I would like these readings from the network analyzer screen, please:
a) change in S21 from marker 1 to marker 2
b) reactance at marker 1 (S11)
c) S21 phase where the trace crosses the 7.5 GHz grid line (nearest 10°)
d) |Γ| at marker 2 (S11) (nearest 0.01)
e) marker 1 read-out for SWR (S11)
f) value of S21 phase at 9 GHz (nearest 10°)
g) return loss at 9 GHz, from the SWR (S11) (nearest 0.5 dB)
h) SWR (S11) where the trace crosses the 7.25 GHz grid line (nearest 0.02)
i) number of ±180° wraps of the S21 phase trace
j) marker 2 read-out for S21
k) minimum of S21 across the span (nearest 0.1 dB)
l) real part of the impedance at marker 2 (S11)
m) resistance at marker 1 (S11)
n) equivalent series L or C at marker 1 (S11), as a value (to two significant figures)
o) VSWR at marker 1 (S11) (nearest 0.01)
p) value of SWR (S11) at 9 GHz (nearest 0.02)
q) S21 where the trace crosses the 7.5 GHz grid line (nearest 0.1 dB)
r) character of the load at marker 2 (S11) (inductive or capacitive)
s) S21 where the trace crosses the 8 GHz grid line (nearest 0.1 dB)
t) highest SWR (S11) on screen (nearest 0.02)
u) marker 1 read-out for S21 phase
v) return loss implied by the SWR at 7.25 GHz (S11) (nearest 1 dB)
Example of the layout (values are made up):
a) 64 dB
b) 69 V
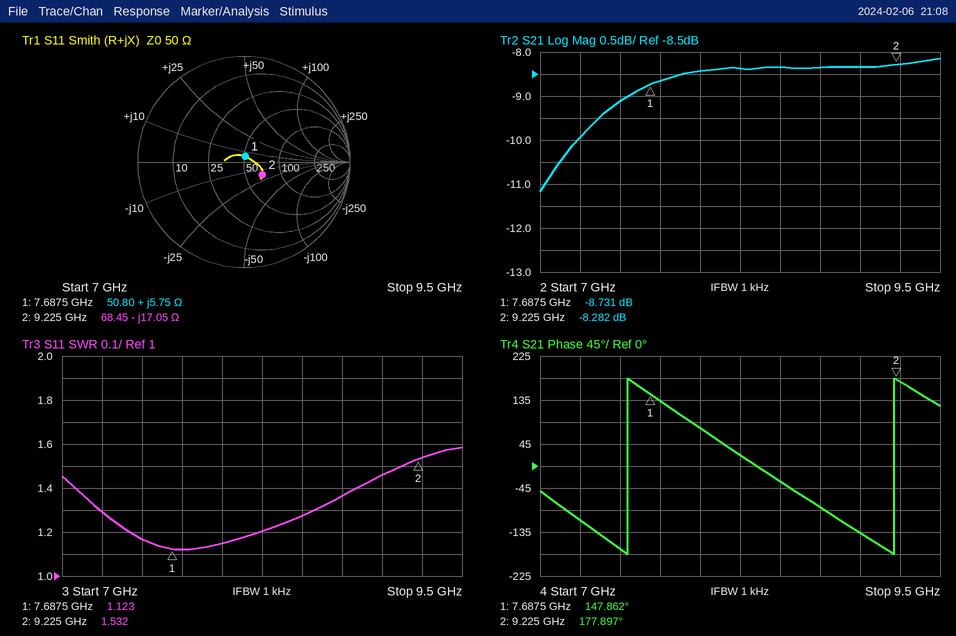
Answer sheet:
a) 0.449 dB
b) +5.75 Ω
c) -170°
d) 0.21
e) 1.123
f) -140°
g) 14.5 dB
h) 1.30
i) 2
j) -8.282 dB
k) -11.2 dB
l) 68.45 Ω
m) 50.80 Ω
n) 120 pH
o) 1.12
p) 1.46
q) -9.1 dB
r) capacitive
s) -8.4 dB
t) 1.58
u) 147.862°
v) 18 dB
